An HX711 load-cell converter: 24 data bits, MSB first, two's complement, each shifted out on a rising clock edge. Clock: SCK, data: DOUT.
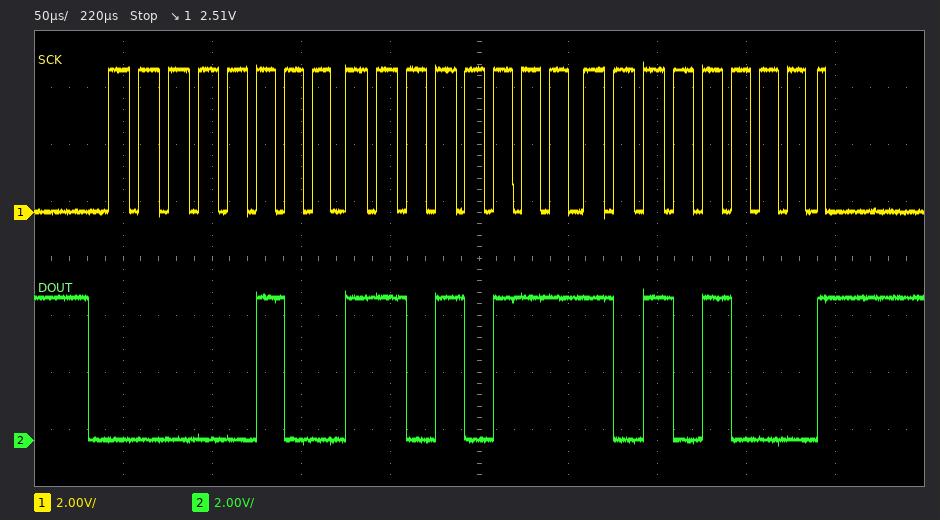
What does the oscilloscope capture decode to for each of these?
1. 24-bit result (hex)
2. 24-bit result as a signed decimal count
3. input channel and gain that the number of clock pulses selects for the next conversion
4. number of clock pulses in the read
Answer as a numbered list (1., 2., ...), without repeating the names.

1. 0x04D7A8
2. 317352
3. channel A, gain 128
4. 25
